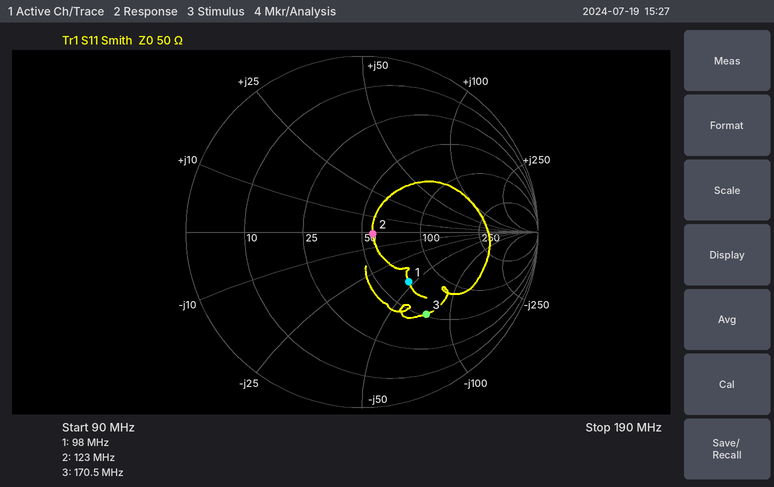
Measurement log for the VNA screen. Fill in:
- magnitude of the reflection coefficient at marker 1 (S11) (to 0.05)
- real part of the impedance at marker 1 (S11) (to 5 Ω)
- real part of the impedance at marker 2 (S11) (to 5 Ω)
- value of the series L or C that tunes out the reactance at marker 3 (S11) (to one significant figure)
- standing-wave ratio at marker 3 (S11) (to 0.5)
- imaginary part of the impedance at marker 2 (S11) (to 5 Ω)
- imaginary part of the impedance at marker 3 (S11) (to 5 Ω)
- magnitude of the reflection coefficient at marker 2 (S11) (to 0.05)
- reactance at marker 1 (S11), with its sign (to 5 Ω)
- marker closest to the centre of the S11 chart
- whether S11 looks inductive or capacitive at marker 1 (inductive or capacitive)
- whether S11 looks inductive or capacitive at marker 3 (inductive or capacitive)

0.40
70 Ω
55 Ω
70 nH
4.0
0 Ω
-75 Ω
0.05
-45 Ω
marker 2
capacitive
capacitive
